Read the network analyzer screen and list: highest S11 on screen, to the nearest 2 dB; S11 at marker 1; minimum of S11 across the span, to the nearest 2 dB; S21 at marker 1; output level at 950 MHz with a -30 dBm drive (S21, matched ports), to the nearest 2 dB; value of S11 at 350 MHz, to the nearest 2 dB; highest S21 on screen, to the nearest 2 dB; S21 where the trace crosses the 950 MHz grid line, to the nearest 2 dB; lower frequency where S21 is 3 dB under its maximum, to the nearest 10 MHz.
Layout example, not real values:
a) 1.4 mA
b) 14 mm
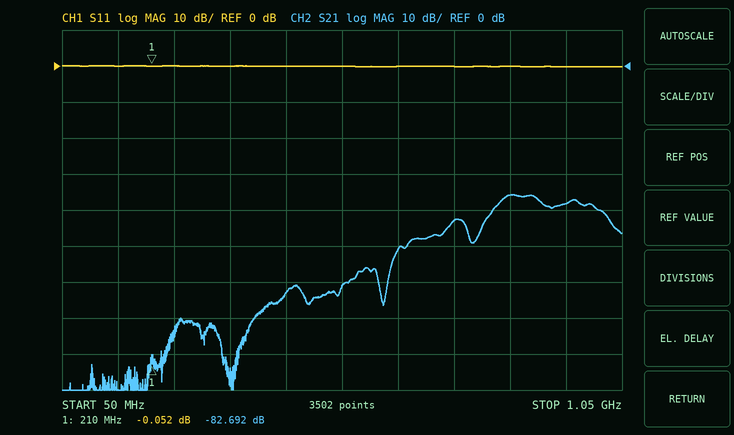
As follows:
a) 0 dB
b) -0.052 dB
c) 0 dB
d) -82.692 dB
e) -68 dBm
f) 0 dB
g) -36 dB
h) -38 dB
i) 830 MHz
